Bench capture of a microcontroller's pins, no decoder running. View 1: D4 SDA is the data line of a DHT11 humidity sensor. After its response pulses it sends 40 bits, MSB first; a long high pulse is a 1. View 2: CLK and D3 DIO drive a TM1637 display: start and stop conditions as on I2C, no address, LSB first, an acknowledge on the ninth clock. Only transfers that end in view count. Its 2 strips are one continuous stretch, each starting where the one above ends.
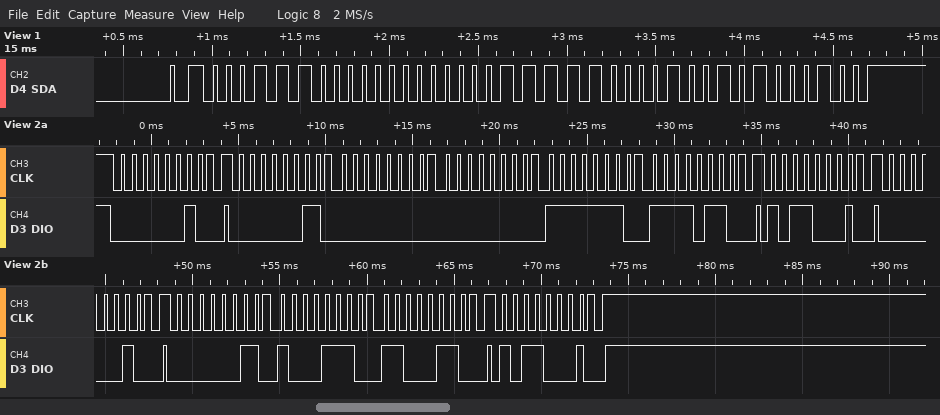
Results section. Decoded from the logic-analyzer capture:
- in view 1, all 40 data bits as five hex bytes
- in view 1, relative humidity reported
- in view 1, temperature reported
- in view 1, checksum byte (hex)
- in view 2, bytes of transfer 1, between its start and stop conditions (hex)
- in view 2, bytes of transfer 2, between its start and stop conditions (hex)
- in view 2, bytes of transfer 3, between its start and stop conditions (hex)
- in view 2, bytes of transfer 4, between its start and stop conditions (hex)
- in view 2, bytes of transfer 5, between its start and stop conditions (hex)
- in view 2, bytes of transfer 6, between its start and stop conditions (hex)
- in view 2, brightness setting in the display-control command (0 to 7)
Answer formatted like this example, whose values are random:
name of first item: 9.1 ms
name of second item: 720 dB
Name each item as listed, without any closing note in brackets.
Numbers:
in view 1, all 40 data bits as five hex bytes: 1C 00 1F 09 44
in view 1, relative humidity reported: 28 %
in view 1, temperature reported: 31.9 °C
in view 1, checksum byte: 0x44
in view 2, bytes of transfer 1, between its start and stop conditions: 40
in view 2, bytes of transfer 2, between its start and stop conditions: C0 00 00 7F 6F
in view 2, bytes of transfer 3, between its start and stop conditions: 8D
in view 2, bytes of transfer 4, between its start and stop conditions: 40
in view 2, bytes of transfer 5, between its start and stop conditions: C0 71 63
in view 2, bytes of transfer 6, between its start and stop conditions: 8D
in view 2, brightness setting in the display-control command: 5
